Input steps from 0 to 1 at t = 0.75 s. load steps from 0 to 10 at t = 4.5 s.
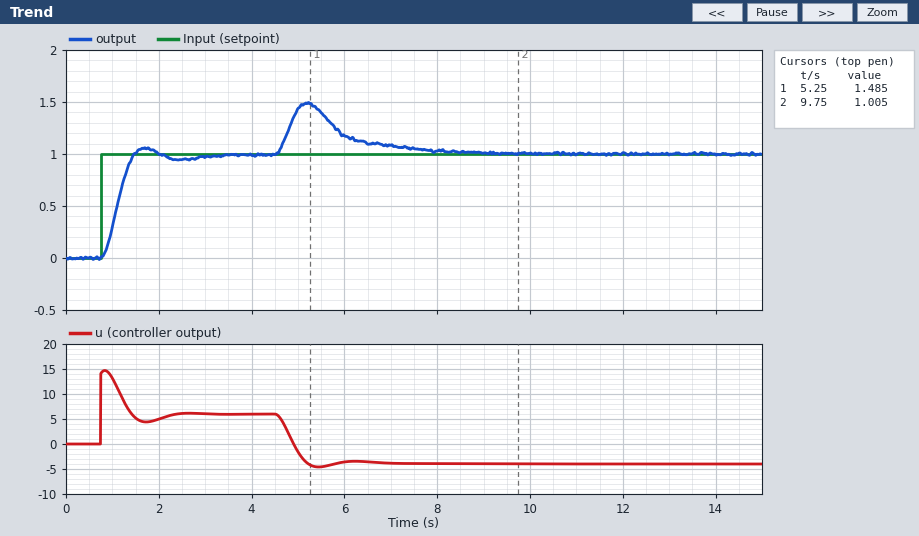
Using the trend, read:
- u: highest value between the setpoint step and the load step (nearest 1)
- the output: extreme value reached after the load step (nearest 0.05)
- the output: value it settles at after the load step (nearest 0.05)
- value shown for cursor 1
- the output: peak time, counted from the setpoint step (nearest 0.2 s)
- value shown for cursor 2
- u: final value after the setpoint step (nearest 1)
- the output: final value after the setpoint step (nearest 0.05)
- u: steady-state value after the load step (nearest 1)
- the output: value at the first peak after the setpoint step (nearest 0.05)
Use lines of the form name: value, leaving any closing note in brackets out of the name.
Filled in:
u: highest value between the setpoint step and the load step: 15
the output: extreme value reached after the load step: 1.50
the output: value it settles at after the load step: 1.00
value shown for cursor 1: 1.485
the output: peak time, counted from the setpoint step: 1.0 s
value shown for cursor 2: 1.005
u: final value after the setpoint step: 6
the output: final value after the setpoint step: 1.00
u: steady-state value after the load step: -4
the output: value at the first peak after the setpoint step: 1.05
